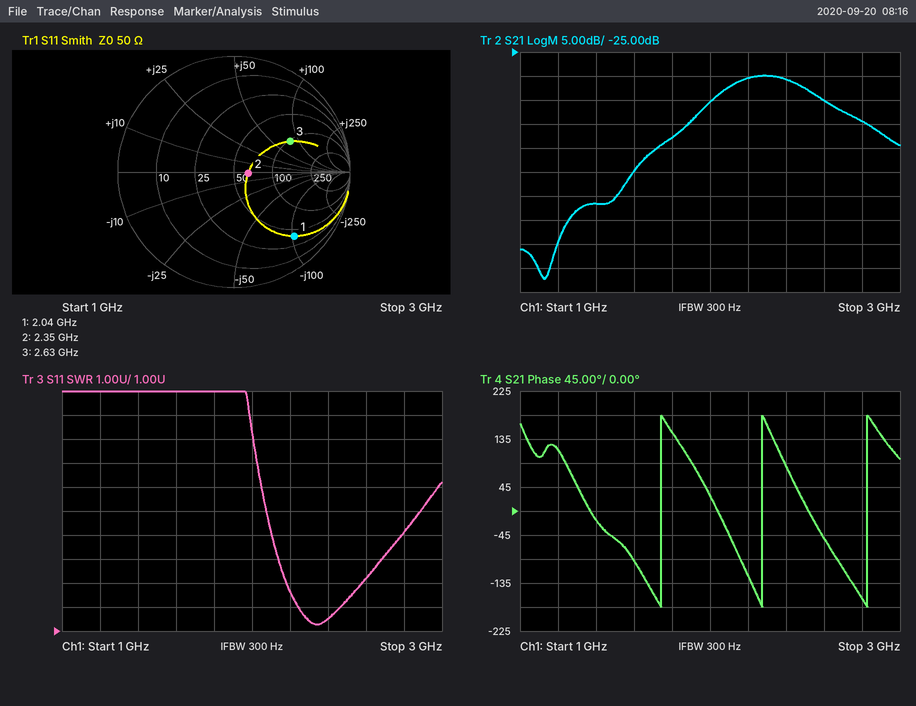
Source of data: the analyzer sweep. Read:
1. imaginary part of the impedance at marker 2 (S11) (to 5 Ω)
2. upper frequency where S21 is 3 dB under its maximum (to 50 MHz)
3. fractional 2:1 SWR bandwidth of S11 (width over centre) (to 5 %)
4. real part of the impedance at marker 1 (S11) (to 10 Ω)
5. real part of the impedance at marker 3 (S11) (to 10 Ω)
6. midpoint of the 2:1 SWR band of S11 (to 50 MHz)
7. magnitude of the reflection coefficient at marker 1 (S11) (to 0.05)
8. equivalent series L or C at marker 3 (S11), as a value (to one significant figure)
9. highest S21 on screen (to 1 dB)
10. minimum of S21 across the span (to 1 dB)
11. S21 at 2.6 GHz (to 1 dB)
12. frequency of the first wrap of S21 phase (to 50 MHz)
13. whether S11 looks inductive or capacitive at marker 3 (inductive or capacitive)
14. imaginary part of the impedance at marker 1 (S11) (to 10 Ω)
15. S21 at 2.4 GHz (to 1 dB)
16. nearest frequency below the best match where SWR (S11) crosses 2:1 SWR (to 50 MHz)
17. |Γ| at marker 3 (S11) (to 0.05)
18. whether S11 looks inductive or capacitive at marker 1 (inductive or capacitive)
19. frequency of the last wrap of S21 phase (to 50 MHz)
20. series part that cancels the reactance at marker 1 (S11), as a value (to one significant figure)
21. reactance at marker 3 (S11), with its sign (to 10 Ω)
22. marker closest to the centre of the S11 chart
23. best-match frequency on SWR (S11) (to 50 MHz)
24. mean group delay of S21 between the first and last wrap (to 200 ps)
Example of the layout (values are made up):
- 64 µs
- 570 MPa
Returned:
- 0 Ω
- 2.50 GHz
- 10 %
- 40 Ω
- 100 Ω
- 2.35 GHz
- 0.75
- 5 nH
- -30 dB
- -72 dB
- -35 dB
- 1.75 GHz
- inductive
- -100 Ω
- -31 dB
- 2.25 GHz
- 0.55
- capacitive
- 2.85 GHz
- 8 nH
- +80 Ω
- marker 2
- 2.35 GHz
- 1.8 ns
